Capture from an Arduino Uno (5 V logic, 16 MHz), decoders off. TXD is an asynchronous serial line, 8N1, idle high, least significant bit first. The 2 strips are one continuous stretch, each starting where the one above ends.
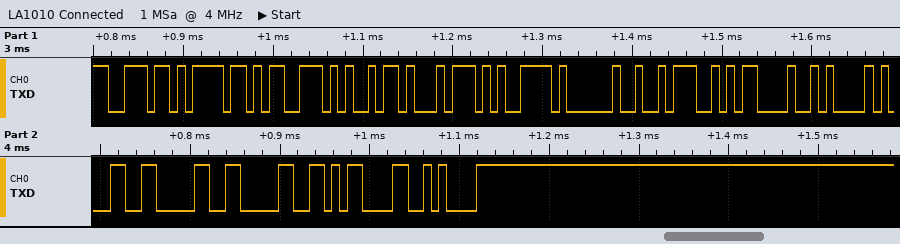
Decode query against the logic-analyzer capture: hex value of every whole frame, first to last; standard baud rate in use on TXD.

6E 6F 73 69 74 79 20 3A 0D 0A 31 30 30 0D 0A
115200 baud
